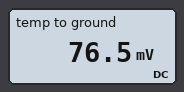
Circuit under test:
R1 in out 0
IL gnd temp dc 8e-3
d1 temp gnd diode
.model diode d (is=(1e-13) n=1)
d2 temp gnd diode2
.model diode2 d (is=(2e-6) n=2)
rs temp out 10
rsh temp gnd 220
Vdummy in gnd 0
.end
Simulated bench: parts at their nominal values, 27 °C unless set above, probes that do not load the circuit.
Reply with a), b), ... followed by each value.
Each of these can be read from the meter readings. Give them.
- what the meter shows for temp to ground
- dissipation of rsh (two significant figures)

a) 76.5 mV
b) 27 µW
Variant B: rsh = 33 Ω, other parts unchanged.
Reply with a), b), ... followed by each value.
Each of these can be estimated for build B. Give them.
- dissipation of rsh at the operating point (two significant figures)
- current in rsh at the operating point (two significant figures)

a) 110 µW
b) 1.9 mA
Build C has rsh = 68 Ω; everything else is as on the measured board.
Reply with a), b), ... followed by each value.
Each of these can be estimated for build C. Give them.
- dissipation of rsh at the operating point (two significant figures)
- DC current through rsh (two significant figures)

a) 71 µW
b) 1.0 mA
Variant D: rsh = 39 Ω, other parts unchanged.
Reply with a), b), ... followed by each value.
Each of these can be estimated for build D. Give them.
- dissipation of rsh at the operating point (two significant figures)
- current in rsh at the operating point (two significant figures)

a) 100 µW
b) 1.6 mA
